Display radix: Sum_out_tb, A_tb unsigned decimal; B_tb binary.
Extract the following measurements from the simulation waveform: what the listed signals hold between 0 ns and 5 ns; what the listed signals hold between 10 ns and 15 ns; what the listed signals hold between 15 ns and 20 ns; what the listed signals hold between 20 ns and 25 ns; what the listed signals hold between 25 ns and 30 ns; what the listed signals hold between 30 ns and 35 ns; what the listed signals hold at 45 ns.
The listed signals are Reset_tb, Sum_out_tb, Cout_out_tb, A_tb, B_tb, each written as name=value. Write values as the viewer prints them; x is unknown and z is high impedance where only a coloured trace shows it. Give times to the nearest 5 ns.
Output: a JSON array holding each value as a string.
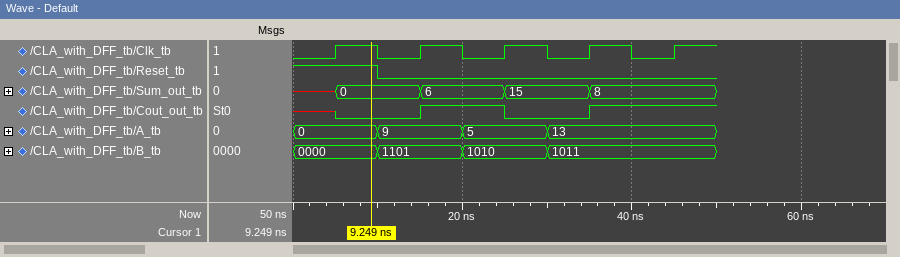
["Reset_tb=1, Sum_out_tb=x, Cout_out_tb=x, A_tb=0, B_tb=0000", "Reset_tb=0, Sum_out_tb=0, Cout_out_tb=0, A_tb=9, B_tb=1101", "Reset_tb=0, Sum_out_tb=6, Cout_out_tb=1, A_tb=9, B_tb=1101", "Reset_tb=0, Sum_out_tb=6, Cout_out_tb=1, A_tb=5, B_tb=1010", "Reset_tb=0, Sum_out_tb=15, Cout_out_tb=0, A_tb=5, B_tb=1010", "Reset_tb=0, Sum_out_tb=15, Cout_out_tb=0, A_tb=13, B_tb=1011", "Reset_tb=0, Sum_out_tb=8, Cout_out_tb=1, A_tb=13, B_tb=1011"]
